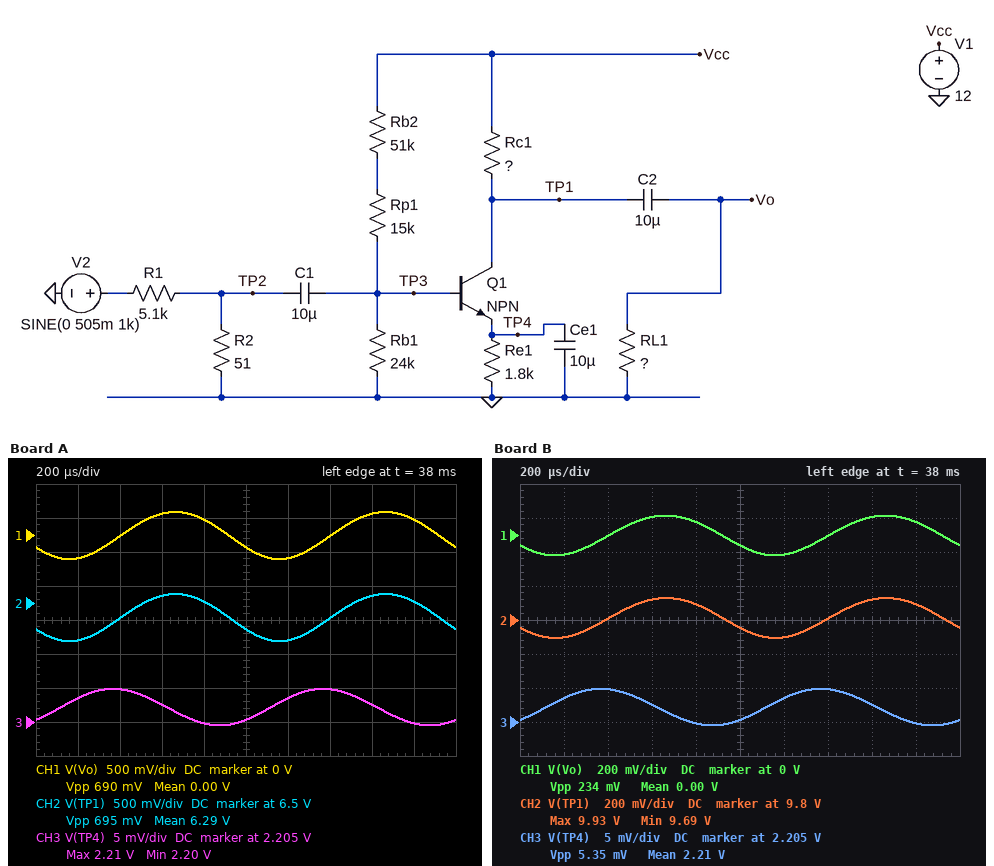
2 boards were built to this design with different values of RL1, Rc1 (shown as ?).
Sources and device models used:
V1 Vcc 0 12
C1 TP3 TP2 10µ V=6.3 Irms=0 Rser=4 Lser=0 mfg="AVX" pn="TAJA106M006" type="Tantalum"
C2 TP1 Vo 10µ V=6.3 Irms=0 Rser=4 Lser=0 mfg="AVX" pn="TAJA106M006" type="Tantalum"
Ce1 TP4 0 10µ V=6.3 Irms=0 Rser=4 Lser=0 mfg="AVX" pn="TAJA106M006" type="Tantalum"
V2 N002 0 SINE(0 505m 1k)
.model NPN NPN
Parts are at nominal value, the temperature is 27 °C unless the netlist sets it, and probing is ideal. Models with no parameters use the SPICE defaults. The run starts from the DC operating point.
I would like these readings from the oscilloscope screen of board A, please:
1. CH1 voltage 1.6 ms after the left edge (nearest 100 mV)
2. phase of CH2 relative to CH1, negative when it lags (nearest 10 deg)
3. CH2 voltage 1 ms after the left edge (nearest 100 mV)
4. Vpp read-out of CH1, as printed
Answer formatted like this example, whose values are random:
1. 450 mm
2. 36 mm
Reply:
1. 300 mV
2. 0 deg
3. 6.1 V
4. 690 mV
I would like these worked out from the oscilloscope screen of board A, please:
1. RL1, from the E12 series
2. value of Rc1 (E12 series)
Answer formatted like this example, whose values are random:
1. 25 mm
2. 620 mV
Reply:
1. 3.9 kΩ
2. 4.7 kΩ
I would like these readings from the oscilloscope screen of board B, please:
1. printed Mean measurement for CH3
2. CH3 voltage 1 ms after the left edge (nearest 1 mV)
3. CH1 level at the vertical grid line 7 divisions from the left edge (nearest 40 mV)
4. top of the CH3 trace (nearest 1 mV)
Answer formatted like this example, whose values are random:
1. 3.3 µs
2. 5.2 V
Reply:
1. 2.21 V
2. 2.205 V
3. 0 V
4. 2.210 V
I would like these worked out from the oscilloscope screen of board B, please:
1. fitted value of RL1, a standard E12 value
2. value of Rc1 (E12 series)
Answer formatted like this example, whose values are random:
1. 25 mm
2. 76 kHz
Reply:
1. 1.2 kΩ
2. 1.8 kΩ
